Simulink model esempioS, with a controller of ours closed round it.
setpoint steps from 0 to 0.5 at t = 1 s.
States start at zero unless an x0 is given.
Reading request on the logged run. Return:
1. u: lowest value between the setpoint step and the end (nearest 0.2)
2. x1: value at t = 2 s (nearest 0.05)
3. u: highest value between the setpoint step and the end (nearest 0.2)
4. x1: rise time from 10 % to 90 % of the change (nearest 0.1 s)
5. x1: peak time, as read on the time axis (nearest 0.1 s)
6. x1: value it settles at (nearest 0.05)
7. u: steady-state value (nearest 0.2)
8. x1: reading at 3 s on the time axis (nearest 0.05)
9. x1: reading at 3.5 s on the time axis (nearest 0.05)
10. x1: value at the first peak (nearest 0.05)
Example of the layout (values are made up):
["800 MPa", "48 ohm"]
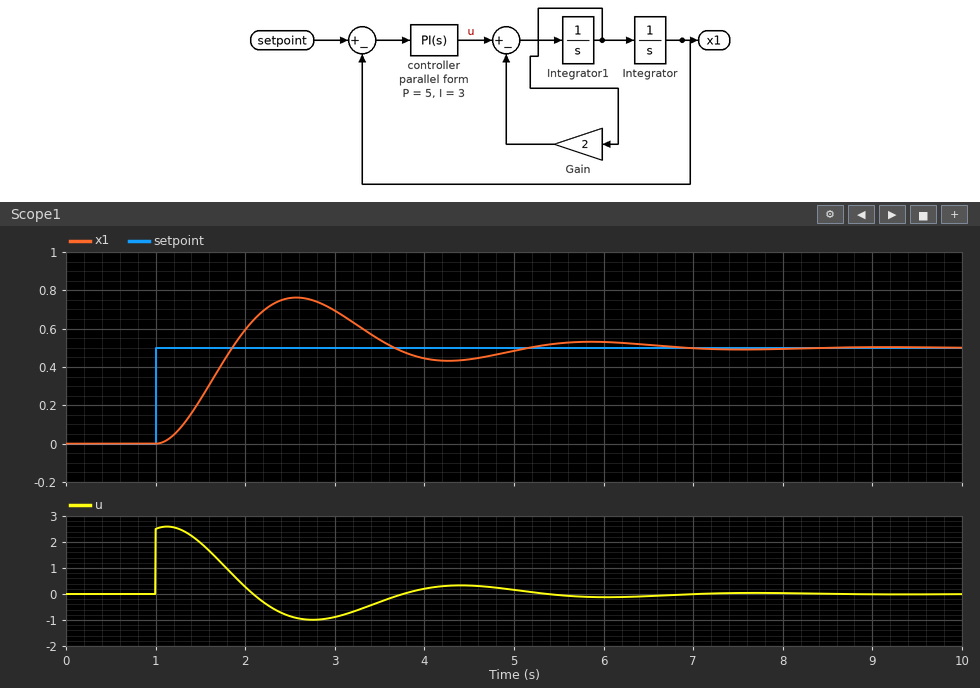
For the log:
["-1.0", "0.60", "2.6", "0.6 s", "2.6 s", "0.50", "0.0", "0.70", "0.55", "0.75"]
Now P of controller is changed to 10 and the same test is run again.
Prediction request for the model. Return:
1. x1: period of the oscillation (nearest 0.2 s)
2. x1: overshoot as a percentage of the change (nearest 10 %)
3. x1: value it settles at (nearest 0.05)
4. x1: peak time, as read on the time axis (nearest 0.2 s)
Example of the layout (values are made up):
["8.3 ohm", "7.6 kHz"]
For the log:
["2.2 s", "50 %", "0.50", "2.0 s"]
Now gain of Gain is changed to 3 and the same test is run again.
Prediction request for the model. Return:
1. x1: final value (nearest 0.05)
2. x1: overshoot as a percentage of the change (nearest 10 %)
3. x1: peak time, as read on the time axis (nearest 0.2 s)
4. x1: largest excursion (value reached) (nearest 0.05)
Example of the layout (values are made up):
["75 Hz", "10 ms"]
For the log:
["0.50", "40 %", "2.8 s", "0.70"]
